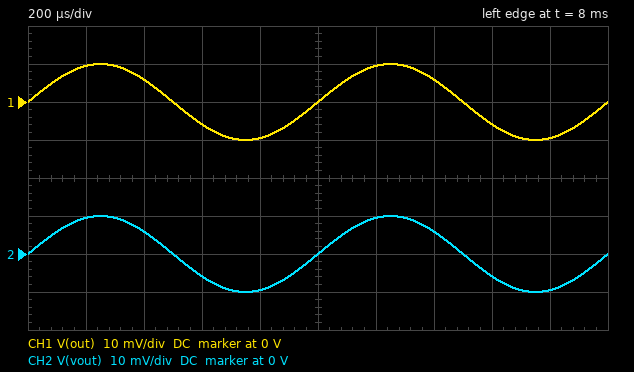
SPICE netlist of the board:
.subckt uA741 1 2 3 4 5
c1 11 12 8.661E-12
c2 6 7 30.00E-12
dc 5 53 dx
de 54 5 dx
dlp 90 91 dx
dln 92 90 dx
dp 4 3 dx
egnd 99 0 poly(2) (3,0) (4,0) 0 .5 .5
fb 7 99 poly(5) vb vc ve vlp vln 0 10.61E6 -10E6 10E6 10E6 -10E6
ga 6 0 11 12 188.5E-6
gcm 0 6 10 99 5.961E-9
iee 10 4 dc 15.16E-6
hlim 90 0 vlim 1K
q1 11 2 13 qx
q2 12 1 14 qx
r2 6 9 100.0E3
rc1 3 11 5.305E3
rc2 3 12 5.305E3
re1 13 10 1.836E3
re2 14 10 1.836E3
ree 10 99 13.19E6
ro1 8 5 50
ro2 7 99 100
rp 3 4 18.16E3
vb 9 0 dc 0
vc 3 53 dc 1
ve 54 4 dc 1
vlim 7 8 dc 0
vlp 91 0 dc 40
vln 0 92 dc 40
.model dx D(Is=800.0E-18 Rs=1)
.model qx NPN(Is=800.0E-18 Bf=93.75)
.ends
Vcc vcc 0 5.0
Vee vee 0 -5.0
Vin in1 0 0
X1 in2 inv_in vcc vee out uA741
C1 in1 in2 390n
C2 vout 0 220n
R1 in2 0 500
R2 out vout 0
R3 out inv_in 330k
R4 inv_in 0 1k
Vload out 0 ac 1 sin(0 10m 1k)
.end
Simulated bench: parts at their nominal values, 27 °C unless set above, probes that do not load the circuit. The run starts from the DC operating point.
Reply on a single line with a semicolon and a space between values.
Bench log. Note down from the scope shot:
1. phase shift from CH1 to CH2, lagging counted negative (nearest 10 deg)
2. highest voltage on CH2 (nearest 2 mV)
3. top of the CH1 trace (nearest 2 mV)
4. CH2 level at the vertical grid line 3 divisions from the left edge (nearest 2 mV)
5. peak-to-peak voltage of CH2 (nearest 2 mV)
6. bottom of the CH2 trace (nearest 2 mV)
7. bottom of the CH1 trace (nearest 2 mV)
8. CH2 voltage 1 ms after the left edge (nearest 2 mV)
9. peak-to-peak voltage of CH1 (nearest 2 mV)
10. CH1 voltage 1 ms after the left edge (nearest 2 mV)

0 deg; 10 mV; 10 mV; -6 mV; 20 mV; -10 mV; -10 mV; 0 V; 20 mV; 0 V
